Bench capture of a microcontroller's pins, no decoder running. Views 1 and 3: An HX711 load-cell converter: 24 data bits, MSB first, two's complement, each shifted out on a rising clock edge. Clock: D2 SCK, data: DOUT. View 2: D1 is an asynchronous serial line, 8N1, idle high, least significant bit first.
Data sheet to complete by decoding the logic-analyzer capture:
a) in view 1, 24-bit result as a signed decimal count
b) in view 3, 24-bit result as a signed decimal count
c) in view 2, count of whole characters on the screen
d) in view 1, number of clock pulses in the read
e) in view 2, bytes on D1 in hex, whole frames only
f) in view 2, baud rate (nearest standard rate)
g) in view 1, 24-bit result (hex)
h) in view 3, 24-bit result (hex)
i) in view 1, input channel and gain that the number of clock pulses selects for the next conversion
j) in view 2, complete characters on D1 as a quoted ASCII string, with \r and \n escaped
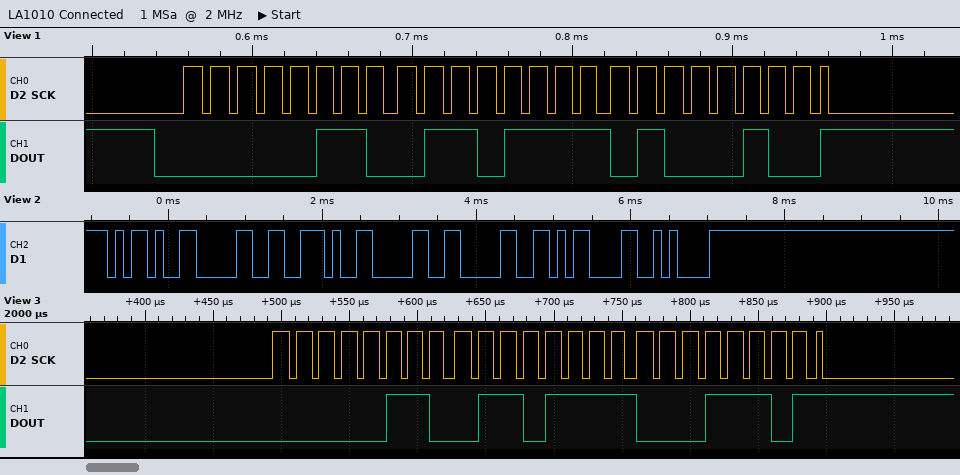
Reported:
421700
421661
7
25
0x2D 0x30 0x2E 0x30 0x30 0x0D 0x0A
9600 baud
0x066F44
0x066F1D
channel A, gain 128
"-0.00\r\n"
